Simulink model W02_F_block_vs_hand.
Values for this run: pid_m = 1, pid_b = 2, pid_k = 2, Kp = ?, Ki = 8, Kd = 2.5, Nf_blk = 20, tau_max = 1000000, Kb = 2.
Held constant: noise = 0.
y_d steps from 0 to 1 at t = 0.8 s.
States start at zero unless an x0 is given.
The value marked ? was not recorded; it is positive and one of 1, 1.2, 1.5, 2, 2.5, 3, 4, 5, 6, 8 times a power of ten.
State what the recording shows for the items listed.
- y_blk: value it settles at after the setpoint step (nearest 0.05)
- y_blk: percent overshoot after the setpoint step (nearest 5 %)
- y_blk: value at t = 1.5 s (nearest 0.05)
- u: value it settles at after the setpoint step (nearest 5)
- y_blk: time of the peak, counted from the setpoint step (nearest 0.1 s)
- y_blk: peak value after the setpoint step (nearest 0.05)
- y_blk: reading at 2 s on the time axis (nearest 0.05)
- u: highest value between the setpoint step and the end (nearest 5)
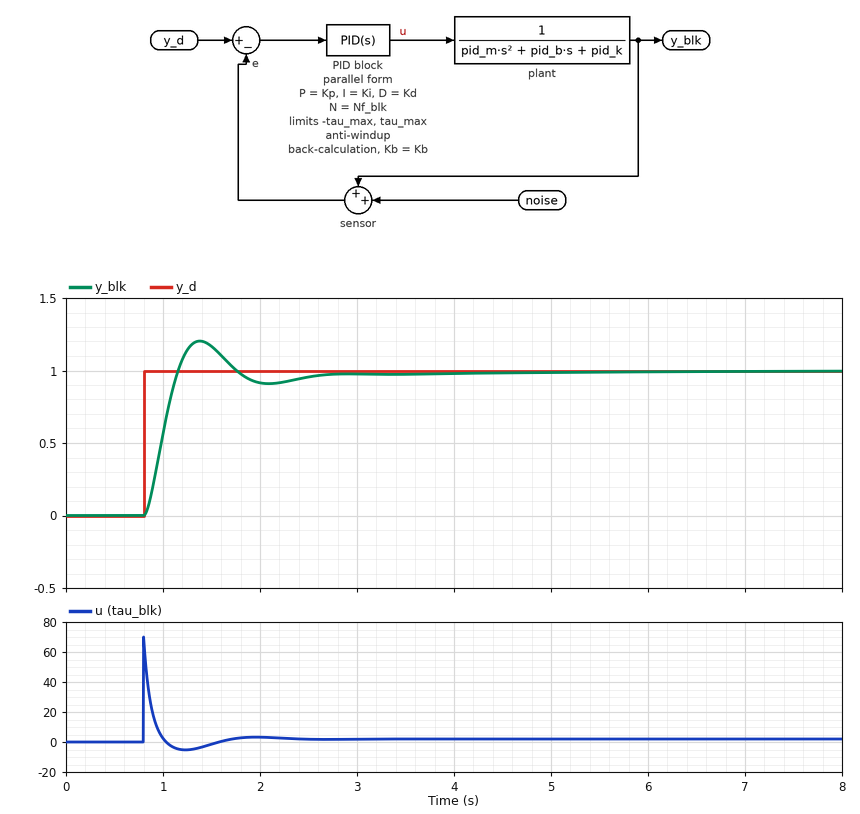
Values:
1.00
20 %
1.15
0
0.6 s
1.20
0.90
70
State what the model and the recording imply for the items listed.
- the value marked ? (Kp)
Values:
20
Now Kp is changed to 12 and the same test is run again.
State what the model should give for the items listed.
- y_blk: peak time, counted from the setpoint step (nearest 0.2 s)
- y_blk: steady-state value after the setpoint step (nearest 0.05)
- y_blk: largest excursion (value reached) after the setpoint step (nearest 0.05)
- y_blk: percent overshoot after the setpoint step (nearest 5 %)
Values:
0.8 s
1.00
1.10
10 %
